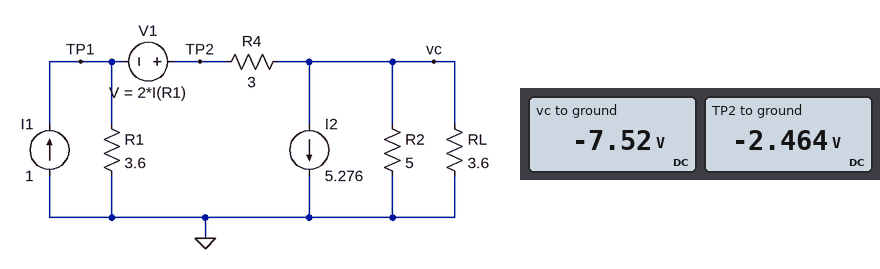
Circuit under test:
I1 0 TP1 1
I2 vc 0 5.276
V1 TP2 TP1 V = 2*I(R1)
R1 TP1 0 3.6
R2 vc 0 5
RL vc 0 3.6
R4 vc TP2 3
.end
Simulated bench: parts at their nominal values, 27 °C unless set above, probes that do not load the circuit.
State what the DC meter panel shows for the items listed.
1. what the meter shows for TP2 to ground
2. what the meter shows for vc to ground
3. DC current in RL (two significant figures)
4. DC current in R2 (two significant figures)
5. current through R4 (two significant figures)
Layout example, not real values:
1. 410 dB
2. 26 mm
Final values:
1. -2.464 V
2. -7.52 V
3. 2.1 A
4. 1.5 A
5. 1.7 A
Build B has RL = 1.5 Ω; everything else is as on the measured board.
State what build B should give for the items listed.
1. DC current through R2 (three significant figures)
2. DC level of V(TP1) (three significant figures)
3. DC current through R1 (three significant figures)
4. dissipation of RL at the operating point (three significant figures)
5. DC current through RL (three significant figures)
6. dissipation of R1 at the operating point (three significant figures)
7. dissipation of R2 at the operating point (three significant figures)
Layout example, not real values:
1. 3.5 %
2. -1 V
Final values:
1. 929 mA
2. -898 mV
3. 249 mA
4. 14.4 W
5. 3.10 A
6. 224 mW
7. 4.32 W
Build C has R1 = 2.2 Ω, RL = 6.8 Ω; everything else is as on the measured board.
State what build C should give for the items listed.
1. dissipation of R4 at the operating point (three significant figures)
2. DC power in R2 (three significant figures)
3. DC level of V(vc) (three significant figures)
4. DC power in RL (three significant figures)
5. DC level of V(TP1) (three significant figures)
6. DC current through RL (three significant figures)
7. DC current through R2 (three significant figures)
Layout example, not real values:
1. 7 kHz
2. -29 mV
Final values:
1. 13.9 W
2. 16.2 W
3. -9.00 V
4. 11.9 W
5. -2.54 V
6. 1.32 A
7. 1.80 A
